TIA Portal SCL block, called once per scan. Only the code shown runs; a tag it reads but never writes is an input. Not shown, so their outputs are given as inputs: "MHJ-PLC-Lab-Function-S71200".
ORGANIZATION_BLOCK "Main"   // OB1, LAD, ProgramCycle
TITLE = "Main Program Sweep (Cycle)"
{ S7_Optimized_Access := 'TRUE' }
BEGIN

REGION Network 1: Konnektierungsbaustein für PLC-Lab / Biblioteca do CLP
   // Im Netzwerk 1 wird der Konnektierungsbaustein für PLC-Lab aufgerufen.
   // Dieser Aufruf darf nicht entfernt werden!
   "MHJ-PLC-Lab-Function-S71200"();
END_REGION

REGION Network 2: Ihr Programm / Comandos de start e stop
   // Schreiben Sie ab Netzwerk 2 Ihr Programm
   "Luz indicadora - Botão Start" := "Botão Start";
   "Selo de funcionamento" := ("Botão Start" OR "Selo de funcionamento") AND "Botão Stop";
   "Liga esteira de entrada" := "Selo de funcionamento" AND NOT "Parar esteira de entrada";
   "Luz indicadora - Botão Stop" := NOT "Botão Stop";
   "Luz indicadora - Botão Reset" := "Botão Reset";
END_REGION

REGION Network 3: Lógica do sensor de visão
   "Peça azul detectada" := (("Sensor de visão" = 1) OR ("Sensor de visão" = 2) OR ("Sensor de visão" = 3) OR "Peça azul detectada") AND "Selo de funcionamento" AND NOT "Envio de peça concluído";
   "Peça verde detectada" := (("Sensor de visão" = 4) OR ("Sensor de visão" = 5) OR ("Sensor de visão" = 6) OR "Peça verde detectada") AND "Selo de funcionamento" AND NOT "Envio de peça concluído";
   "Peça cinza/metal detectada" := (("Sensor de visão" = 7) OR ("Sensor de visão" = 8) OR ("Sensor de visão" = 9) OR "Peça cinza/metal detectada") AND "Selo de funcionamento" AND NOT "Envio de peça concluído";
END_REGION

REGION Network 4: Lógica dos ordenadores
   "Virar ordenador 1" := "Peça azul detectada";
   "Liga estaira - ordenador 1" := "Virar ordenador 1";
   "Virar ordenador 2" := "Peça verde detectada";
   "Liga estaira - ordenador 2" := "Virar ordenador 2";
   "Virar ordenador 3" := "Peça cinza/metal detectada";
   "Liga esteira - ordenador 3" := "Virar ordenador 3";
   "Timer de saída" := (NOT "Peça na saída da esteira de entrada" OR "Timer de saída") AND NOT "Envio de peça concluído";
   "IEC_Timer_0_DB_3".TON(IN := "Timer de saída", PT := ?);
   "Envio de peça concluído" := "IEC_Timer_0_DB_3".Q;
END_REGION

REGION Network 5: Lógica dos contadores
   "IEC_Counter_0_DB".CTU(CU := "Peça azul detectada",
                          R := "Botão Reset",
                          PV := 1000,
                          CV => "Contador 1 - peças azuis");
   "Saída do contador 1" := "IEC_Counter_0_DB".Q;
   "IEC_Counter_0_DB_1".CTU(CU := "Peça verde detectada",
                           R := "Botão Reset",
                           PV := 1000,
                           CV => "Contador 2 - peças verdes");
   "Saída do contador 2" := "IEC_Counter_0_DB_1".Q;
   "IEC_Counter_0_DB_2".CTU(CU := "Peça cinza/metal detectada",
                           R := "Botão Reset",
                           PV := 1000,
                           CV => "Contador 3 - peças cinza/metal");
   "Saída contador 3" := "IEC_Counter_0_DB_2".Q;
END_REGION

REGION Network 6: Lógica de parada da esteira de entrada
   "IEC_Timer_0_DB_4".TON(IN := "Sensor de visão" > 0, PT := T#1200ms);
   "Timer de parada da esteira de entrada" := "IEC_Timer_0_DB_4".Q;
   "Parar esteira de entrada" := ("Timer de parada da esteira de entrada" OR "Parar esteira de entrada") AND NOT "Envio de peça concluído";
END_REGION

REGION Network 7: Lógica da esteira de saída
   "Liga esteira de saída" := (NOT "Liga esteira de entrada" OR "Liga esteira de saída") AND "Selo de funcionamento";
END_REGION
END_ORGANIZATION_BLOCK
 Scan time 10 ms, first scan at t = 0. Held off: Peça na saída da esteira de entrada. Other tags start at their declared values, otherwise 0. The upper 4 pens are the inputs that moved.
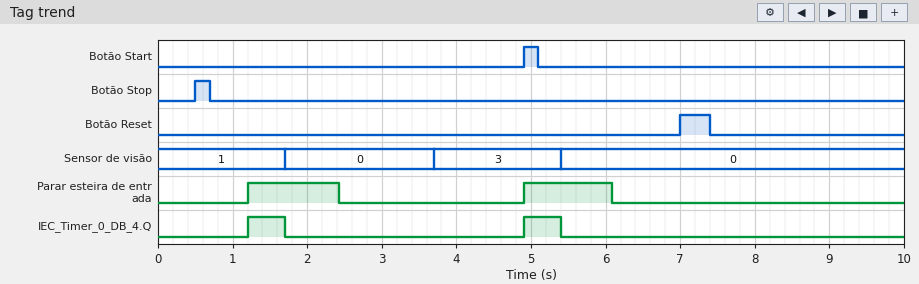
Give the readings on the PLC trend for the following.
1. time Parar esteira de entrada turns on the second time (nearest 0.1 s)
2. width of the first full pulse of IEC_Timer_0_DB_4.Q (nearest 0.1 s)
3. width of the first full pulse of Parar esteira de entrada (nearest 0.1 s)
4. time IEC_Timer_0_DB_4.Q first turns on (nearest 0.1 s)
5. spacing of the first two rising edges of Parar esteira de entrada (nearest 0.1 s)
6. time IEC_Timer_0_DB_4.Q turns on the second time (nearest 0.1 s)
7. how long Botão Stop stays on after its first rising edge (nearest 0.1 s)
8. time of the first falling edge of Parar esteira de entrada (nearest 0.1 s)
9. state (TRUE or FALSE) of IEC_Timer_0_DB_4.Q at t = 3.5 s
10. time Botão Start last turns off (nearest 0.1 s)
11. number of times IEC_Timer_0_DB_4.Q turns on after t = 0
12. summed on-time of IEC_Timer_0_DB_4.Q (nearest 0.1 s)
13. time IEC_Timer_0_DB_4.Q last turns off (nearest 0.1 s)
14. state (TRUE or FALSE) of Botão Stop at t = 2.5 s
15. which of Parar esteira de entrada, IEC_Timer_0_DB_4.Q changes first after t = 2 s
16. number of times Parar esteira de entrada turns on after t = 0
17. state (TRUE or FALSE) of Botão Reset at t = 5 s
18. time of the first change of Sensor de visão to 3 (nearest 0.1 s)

4.9 s
0.5 s
1.2 s
1.2 s
3.7 s
4.9 s
0.2 s
2.4 s
FALSE
5.1 s
2
1.0 s
5.4 s
FALSE
Parar esteira de entrada
2
FALSE
3.7 s
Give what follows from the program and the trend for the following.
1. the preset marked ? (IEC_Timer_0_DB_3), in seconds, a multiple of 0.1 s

1.2 s
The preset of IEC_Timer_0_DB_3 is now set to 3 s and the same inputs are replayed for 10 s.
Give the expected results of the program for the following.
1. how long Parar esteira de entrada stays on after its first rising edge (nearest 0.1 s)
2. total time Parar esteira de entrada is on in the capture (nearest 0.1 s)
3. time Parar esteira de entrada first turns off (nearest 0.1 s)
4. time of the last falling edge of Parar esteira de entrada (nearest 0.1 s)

1.8 s
2.9 s
3.0 s
6.0 s
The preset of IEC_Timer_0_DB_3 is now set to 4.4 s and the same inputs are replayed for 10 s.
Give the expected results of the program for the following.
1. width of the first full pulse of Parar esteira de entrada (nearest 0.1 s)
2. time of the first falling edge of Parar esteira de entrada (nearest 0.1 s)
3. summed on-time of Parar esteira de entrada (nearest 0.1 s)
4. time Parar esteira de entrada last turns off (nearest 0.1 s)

3.2 s
4.4 s
7.1 s
8.8 s
